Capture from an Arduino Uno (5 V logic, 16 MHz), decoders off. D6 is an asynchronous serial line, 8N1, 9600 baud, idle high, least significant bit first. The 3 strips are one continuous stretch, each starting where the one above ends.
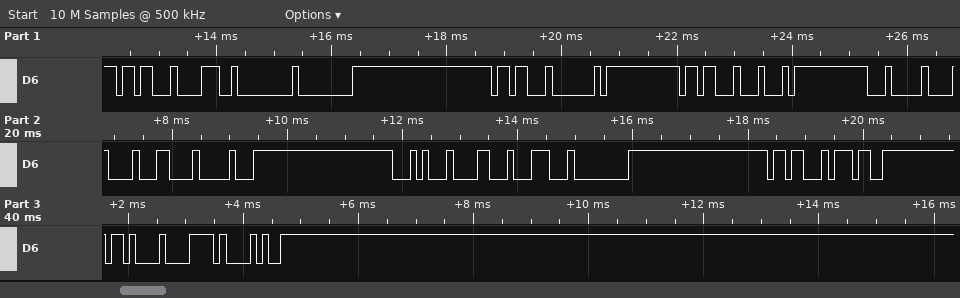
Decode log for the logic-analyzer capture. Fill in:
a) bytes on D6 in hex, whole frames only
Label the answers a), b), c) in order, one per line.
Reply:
a) 0x1B 0x38 0x00 0x00 0x1B 0x40 0x1B 0x44 0x04 0x08 0x0C 0x10 0x14 0x18 0x1C 0x00 0x1B 0x37 0x0B 0x78 0x28
